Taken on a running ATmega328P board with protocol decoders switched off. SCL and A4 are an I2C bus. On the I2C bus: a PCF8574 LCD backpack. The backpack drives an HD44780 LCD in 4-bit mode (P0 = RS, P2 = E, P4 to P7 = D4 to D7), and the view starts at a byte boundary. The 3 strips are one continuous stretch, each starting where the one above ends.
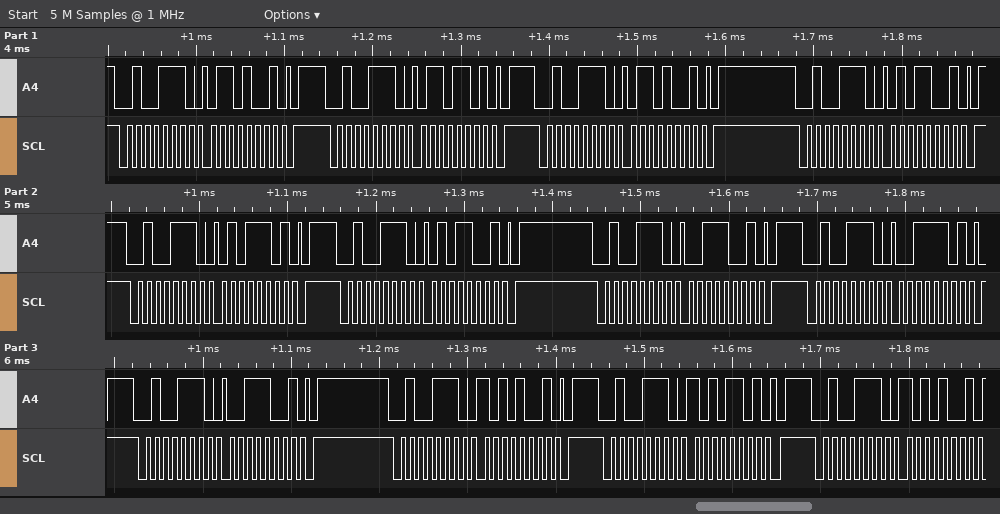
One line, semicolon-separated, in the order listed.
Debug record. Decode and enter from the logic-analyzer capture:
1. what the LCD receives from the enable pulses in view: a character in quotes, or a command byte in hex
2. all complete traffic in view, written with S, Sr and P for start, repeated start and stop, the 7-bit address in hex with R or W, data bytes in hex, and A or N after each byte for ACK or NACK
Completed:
'e' ':'; S 27W A 69 A P S 27W A 6D A P S 27W A 69 A P S 27W A 59 A P S 27W A 5D A P S 27W A 59 A P S 27W A 39 A P S 27W A 3D A P S 27W A 39 A P S 27W A A9 A P S 27W A AD A P S 27W A A9 A
